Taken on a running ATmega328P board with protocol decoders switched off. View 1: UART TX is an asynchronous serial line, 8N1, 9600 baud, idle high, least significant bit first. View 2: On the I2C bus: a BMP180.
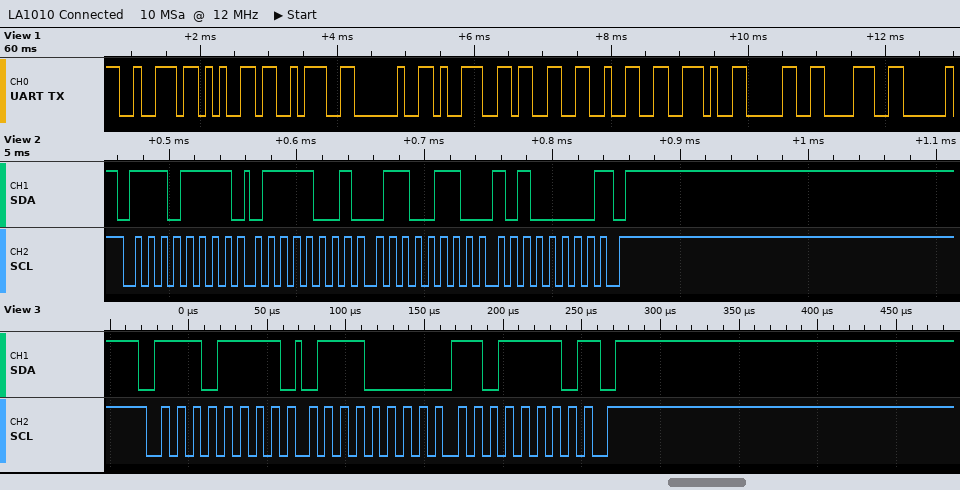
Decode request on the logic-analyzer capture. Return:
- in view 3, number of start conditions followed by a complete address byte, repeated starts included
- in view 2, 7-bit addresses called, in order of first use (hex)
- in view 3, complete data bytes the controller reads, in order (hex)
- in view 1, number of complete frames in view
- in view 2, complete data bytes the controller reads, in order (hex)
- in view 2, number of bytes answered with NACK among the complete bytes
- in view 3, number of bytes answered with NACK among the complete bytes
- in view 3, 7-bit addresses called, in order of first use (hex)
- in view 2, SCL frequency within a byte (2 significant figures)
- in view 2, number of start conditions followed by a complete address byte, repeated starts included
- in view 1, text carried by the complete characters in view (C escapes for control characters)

1
0x77
70 DE
10
79 66 A0
1
1
0x77
100 kHz
1
"re: 932.08"
